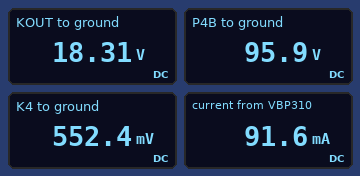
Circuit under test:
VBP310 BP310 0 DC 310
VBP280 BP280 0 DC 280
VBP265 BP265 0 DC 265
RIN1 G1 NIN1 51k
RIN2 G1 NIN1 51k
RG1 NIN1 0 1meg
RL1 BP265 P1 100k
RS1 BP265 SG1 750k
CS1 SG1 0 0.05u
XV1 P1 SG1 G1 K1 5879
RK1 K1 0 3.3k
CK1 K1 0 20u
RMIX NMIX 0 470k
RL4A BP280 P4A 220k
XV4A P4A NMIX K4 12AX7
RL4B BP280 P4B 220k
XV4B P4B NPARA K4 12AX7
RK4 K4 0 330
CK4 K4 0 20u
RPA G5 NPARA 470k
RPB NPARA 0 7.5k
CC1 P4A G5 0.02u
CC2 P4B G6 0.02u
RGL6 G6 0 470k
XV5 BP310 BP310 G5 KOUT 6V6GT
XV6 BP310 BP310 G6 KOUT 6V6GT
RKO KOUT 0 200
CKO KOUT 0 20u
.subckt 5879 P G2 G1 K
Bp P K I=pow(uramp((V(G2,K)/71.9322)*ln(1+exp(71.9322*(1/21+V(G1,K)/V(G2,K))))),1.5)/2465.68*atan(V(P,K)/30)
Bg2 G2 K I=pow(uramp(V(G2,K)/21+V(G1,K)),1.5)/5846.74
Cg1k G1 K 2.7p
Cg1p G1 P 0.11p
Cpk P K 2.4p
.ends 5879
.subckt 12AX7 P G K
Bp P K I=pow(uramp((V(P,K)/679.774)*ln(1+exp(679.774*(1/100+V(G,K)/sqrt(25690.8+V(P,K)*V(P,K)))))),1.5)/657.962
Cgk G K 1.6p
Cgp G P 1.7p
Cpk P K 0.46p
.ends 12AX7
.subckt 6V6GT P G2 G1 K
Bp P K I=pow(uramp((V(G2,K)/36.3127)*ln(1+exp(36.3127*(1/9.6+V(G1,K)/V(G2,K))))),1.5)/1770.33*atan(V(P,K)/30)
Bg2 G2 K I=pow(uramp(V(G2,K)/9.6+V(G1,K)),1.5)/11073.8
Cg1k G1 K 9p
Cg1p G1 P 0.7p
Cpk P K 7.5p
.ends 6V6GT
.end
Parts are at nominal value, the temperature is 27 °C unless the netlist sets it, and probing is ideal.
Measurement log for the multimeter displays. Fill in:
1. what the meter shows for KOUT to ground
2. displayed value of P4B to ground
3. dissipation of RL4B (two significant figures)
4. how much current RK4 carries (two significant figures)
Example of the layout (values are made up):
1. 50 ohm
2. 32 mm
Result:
1. 18.31 V
2. 95.9 V
3. 150 mW
4. 1.7 mA
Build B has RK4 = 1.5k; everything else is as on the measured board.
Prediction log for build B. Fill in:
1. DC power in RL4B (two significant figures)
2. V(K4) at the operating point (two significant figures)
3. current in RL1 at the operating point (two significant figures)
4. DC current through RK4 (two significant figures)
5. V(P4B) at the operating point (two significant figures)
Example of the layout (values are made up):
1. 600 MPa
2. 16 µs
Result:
1. 63 mW
2. 1.6 V
3. 1.3 mA
4. 1.1 mA
5. 160 V
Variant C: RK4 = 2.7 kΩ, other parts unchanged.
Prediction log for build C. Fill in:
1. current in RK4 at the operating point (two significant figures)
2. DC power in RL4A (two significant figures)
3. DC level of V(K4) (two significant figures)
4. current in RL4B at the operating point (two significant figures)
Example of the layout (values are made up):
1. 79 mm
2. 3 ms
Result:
1. 770 µA
2. 33 mW
3. 2.1 V
4. 390 µA
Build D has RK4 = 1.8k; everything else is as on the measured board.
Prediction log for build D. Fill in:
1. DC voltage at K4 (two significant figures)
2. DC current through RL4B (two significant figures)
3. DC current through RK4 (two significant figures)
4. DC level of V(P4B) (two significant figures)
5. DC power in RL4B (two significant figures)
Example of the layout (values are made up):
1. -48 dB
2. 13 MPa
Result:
1. 1.8 V
2. 490 µA
3. 980 µA
4. 170 V
5. 52 mW
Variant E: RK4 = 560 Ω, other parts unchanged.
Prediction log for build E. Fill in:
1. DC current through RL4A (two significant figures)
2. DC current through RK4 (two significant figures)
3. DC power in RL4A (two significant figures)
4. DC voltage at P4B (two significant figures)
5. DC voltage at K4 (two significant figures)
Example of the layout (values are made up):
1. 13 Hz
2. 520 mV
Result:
1. 760 µA
2. 1.5 mA
3. 130 mW
4. 110 V
5. 850 mV
